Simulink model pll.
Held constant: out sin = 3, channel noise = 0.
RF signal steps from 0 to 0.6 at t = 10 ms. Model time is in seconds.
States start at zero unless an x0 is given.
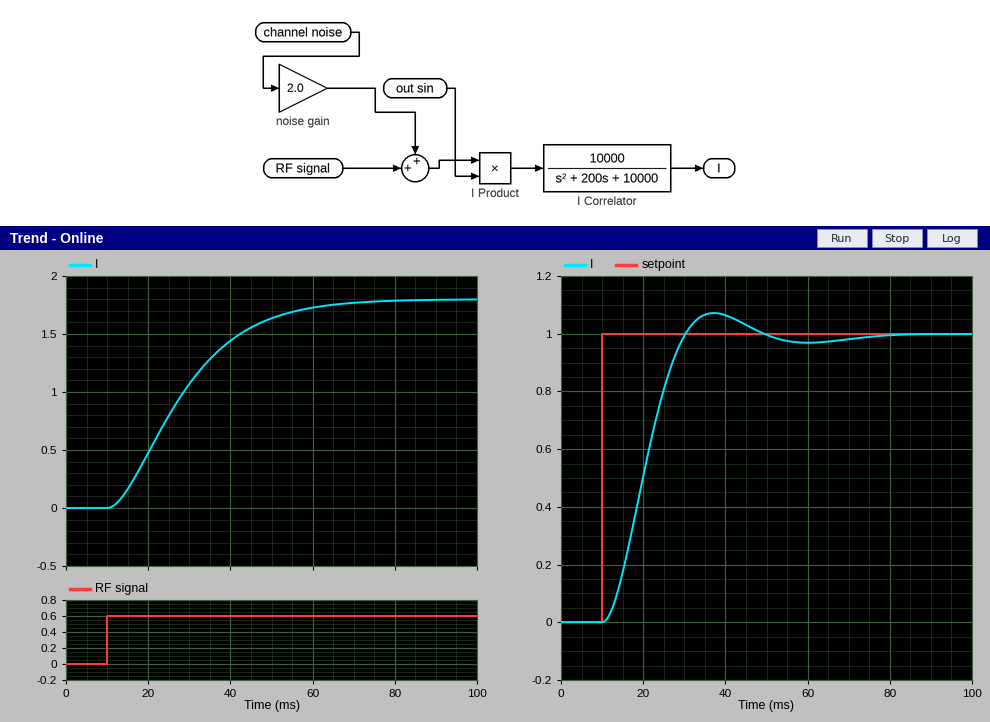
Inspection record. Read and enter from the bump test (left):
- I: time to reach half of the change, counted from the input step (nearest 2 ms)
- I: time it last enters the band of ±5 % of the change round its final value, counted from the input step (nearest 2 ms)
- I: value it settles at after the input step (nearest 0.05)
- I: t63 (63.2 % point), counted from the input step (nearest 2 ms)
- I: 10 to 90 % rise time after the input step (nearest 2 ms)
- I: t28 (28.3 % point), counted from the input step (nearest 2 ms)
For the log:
16 ms
48 ms
1.80
22 ms
34 ms
10 ms
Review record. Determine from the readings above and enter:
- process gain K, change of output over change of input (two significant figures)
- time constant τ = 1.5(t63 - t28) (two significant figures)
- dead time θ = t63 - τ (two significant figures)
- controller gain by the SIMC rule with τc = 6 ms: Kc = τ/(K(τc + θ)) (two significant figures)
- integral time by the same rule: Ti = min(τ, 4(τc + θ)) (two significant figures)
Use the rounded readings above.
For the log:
3.0
18 ms
4.0 ms
0.60
18 ms
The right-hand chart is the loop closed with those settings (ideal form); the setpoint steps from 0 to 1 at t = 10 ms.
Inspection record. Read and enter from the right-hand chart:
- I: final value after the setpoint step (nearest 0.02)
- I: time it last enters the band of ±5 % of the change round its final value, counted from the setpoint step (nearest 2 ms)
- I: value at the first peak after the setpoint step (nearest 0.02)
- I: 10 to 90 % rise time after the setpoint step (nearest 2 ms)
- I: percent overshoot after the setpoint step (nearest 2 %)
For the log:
1.00
32 ms
1.08
14 ms
8 %
